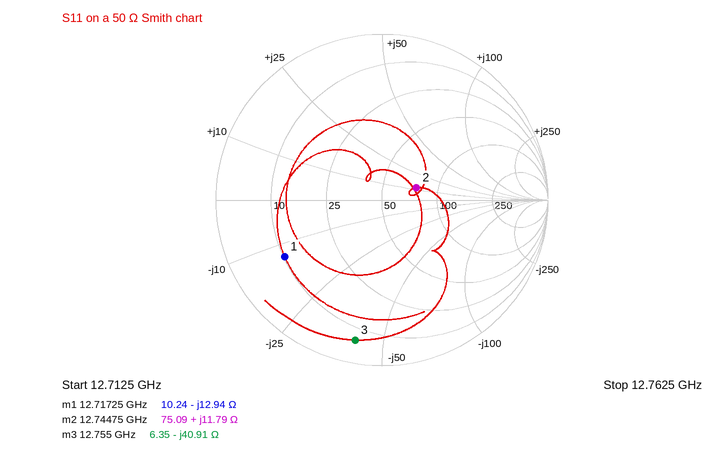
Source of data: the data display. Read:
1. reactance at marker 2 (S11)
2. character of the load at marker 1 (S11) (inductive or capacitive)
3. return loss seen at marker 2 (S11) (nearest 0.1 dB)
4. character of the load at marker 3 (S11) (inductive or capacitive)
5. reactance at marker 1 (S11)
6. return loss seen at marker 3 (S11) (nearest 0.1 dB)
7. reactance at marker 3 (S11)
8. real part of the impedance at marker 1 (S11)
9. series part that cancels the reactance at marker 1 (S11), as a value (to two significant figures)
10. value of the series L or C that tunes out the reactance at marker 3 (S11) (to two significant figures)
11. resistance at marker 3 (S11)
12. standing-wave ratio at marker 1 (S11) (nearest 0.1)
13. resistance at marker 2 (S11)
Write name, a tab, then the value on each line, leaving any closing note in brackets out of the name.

reactance at marker 2	+11.79 Ω
character of the load at marker 1 (S11)	capacitive
return loss seen at marker 2 (S11)	13.1 dB
character of the load at marker 3 (S11)	capacitive
reactance at marker 1	-12.94 Ω
return loss seen at marker 3 (S11)	1.3 dB
reactance at marker 3	-40.91 Ω
real part of the impedance at marker 1	10.24 Ω
series part that cancels the reactance at marker 1 (S11), as a value	160 pH
value of the series L or C that tunes out the reactance at marker 3 (S11)	510 pH
resistance at marker 3	6.35 Ω
standing-wave ratio at marker 1 (S11)	5.2
resistance at marker 2	75.09 Ω
